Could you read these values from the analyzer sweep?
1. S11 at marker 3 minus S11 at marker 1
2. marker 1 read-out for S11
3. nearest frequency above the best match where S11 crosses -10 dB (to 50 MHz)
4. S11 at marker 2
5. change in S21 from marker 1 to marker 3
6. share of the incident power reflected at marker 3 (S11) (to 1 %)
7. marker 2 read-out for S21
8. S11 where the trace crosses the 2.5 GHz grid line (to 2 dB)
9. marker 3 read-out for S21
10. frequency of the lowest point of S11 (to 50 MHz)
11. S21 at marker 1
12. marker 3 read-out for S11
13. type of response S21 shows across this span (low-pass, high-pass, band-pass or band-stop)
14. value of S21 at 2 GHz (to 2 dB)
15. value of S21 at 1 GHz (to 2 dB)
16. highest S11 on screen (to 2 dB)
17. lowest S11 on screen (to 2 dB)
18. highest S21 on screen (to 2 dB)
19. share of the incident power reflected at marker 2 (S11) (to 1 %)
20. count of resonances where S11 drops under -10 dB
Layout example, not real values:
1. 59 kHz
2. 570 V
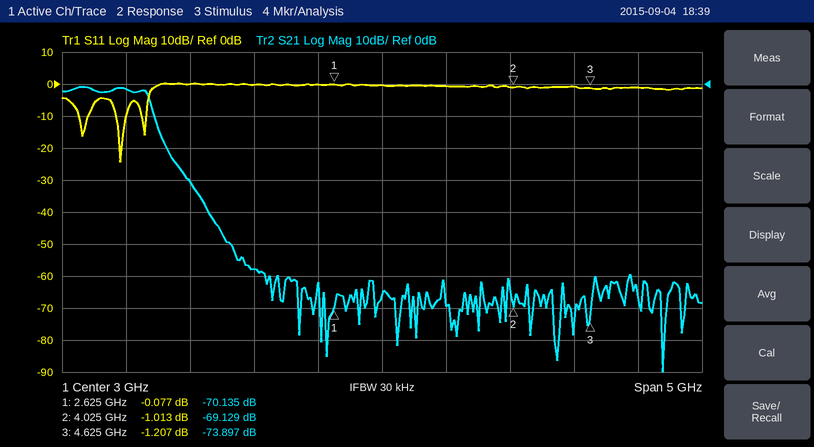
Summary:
1. -1.130 dB
2. -0.077 dB
3. 1.00 GHz
4. -1.013 dB
5. -3.762 dB
6. 76 %
7. -69.129 dB
8. 0 dB
9. -73.897 dB
10. 950 MHz
11. -70.135 dB
12. -1.207 dB
13. low-pass
14. -58 dB
15. -2 dB
16. 0 dB
17. -24 dB
18. 0 dB
19. 79 %
20. 3
